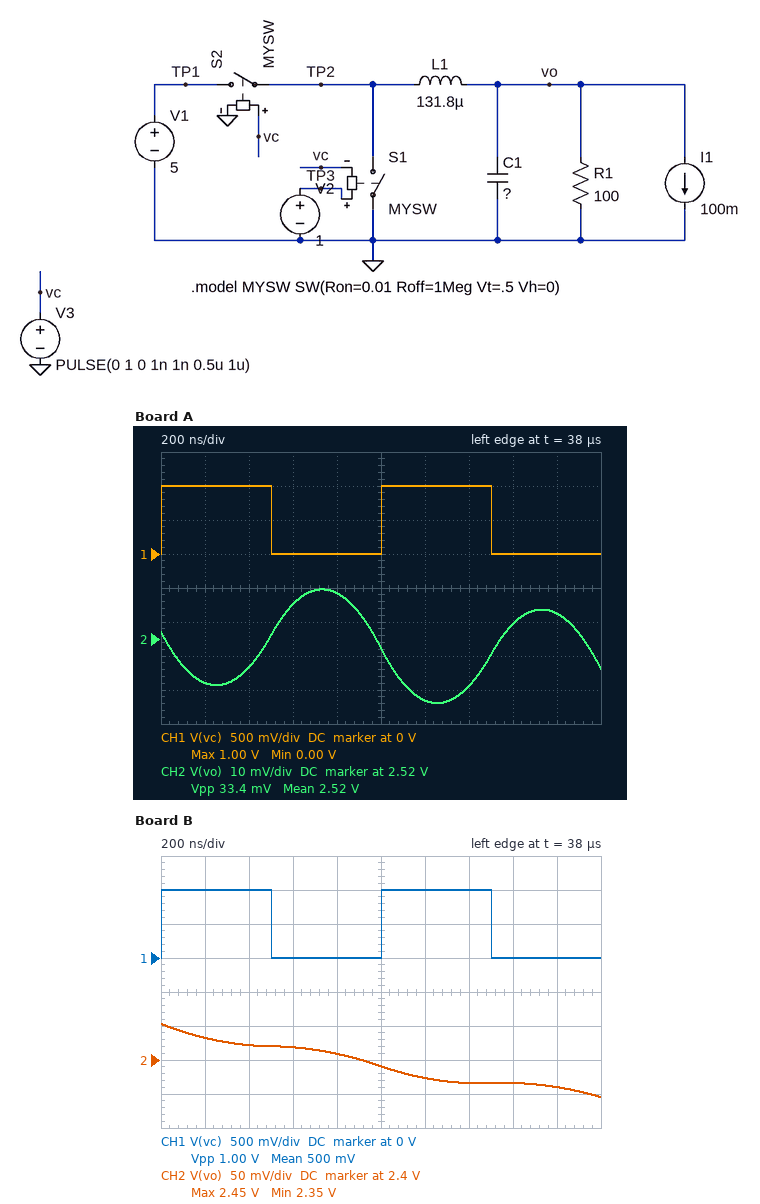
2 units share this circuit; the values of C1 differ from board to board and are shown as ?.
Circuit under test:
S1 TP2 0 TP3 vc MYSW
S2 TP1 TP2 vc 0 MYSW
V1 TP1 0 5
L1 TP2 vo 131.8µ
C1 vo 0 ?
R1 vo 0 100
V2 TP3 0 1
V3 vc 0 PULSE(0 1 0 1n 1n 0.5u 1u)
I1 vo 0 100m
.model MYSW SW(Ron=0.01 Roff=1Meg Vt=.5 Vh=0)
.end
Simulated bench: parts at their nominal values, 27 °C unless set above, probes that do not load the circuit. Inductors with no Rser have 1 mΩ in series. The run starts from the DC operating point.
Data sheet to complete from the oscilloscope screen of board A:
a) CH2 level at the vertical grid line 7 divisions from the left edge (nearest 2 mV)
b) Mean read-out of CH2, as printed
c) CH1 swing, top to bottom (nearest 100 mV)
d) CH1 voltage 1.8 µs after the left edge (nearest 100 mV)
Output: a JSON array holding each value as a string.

["2.506 V", "2.52 V", "1.0 V", "0 V"]
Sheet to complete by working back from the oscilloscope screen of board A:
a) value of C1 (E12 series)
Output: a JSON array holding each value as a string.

["39 nF"]
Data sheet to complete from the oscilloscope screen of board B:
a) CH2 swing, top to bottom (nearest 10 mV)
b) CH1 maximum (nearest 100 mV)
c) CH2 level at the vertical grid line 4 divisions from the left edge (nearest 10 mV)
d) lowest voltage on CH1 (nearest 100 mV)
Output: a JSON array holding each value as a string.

["110 mV", "1.0 V", "2.41 V", "0 V"]
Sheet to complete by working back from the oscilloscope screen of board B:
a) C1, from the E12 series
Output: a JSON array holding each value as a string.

["82 nF"]
